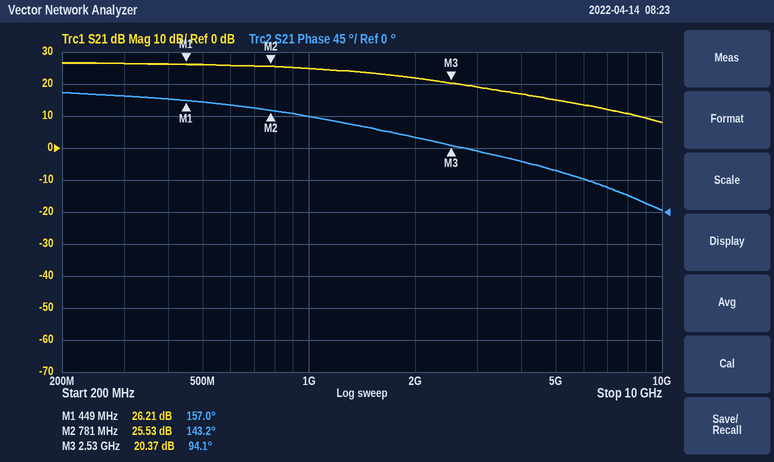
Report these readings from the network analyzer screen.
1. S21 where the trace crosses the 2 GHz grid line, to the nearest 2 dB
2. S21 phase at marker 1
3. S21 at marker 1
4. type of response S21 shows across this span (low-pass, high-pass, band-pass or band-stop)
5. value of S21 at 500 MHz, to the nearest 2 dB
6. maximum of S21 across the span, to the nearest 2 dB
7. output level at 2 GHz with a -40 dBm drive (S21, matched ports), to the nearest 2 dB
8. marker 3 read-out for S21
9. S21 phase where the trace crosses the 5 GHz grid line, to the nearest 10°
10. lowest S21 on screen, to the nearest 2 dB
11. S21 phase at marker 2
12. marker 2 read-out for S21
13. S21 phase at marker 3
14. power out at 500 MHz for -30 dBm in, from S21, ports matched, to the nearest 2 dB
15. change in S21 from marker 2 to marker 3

22 dB
157.0°
26.21 dB
low-pass
26 dB
26 dB
-18 dBm
20.37 dB
60°
8 dB
143.2°
25.53 dB
94.1°
-4 dBm
-5.16 dB
